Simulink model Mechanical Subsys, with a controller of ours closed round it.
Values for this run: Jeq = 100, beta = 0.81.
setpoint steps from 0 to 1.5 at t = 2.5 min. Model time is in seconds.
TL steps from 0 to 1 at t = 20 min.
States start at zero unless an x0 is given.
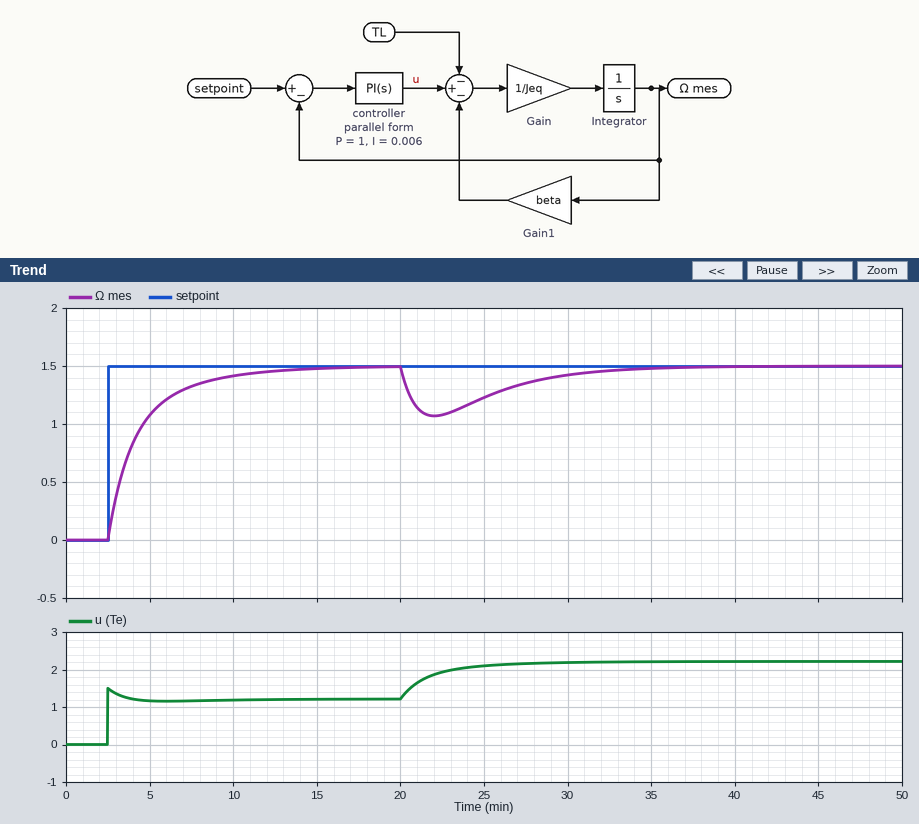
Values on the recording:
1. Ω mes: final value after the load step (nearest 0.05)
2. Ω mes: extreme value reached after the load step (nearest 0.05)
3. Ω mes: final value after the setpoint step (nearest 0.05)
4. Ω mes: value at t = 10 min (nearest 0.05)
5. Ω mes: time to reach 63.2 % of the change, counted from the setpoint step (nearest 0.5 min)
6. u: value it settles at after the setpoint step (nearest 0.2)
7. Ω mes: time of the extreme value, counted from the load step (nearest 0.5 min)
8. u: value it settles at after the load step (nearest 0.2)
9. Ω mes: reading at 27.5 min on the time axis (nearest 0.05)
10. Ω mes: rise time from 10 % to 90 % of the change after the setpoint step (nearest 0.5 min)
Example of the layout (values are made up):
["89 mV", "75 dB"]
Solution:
["1.50", "1.05", "1.50", "1.40", "2.0 min", "1.2", "2.0 min", "2.2", "1.35", "5.5 min"]
